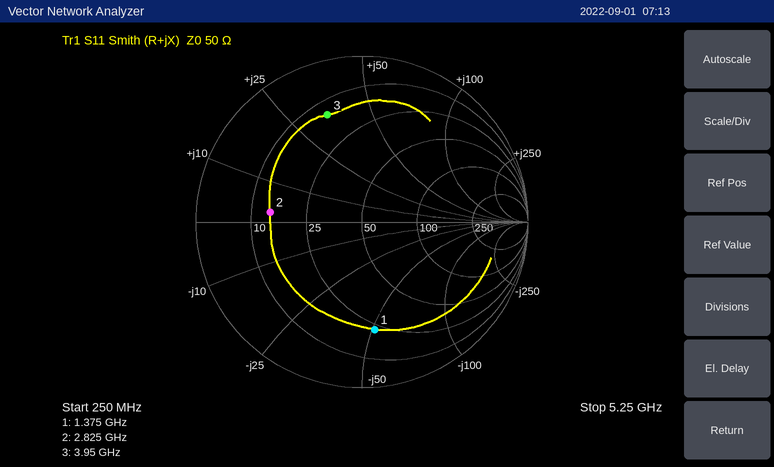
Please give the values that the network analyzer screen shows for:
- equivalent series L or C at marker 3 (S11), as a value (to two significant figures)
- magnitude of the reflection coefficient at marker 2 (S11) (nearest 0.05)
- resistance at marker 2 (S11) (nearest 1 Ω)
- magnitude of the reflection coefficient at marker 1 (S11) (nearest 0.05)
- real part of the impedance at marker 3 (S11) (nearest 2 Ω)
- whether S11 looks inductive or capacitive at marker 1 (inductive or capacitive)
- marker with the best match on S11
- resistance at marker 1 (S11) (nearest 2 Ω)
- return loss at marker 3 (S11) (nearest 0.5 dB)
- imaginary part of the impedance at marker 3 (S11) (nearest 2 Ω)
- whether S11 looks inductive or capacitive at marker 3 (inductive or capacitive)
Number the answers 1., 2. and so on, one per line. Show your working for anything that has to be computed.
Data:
1. L = 34 Ω/(2π × 3.95 GHz) ≈ 1.4 nH
2. 0.55
3. 14 Ω
4. 0.65
5. 14 Ω
6. capacitive
7. marker 2
8. 22 Ω
9. 3.5 dB
10. +34 Ω
11. inductive
